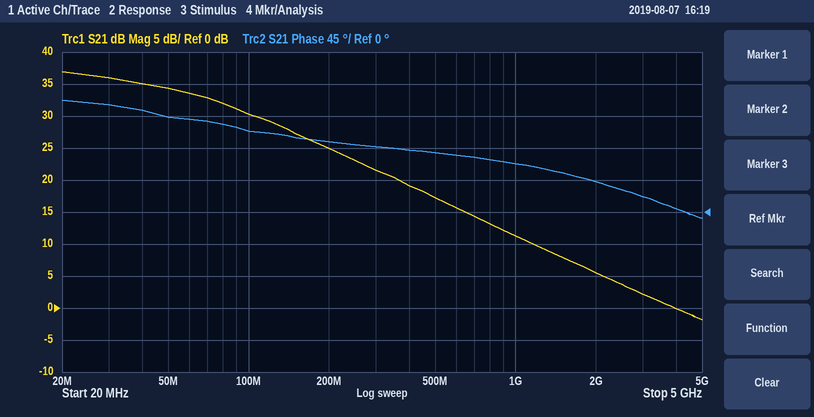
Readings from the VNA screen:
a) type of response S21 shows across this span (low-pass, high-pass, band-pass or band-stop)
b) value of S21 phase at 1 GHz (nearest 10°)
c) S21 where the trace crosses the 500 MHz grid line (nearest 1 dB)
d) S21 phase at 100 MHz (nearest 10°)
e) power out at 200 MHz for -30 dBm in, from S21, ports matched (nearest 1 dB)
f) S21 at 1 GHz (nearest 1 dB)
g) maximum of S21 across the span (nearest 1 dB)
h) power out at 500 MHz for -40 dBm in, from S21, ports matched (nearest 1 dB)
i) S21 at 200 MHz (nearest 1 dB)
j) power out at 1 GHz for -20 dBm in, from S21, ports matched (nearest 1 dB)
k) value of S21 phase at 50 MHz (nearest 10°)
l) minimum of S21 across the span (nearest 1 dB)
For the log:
low-pass
70°
17 dB
110°
-5 dBm
11 dB
37 dB
-23 dBm
25 dB
-9 dBm
130°
-2 dB
